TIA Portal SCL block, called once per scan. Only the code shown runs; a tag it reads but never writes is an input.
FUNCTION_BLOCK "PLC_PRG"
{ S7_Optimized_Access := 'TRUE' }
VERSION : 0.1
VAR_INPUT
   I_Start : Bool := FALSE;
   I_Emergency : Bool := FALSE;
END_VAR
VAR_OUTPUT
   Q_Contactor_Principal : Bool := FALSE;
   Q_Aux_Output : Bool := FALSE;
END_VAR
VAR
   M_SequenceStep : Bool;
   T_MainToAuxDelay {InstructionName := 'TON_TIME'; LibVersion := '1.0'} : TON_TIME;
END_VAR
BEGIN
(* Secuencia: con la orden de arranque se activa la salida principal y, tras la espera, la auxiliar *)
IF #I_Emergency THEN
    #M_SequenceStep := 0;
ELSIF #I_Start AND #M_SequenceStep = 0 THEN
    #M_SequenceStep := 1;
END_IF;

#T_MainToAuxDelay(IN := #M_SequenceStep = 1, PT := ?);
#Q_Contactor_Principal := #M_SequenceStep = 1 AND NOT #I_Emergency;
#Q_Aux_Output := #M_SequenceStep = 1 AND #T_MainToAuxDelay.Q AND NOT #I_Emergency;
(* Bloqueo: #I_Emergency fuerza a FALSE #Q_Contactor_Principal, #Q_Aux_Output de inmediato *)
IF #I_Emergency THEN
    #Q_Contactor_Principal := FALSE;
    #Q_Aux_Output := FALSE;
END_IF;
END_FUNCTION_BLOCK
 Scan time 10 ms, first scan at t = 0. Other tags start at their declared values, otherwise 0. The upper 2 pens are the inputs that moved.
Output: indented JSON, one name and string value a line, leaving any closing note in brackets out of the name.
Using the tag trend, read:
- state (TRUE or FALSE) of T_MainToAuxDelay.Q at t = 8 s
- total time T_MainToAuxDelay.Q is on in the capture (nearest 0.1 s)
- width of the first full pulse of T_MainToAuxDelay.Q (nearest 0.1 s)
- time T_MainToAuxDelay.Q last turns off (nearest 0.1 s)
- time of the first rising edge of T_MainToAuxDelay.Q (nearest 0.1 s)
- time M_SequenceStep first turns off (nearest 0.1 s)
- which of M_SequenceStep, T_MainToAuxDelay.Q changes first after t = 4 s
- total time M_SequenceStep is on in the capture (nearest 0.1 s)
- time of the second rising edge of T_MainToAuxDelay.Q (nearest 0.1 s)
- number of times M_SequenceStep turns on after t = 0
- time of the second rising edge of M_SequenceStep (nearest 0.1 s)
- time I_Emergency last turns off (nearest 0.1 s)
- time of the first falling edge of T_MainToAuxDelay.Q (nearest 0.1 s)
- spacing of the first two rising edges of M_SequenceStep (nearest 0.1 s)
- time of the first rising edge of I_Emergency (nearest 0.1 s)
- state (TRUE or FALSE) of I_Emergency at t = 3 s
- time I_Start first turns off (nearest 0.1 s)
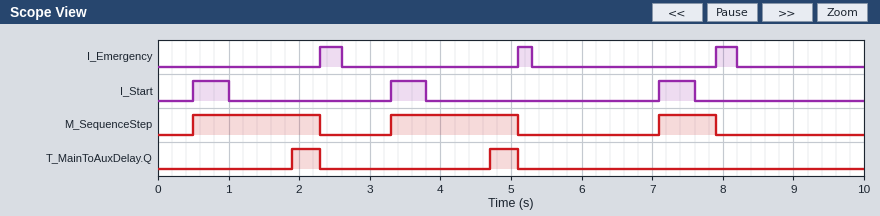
{
  "state (TRUE or FALSE) of T_MainToAuxDelay.Q at t = 8 s": "FALSE",
  "total time T_MainToAuxDelay.Q is on in the capture": "0.8 s",
  "width of the first full pulse of T_MainToAuxDelay.Q": "0.4 s",
  "time T_MainToAuxDelay.Q last turns off": "5.1 s",
  "time of the first rising edge of T_MainToAuxDelay.Q": "1.9 s",
  "time M_SequenceStep first turns off": "2.3 s",
  "which of M_SequenceStep, T_MainToAuxDelay.Q changes first after t = 4 s": "T_MainToAuxDelay.Q",
  "total time M_SequenceStep is on in the capture": "4.4 s",
  "time of the second rising edge of T_MainToAuxDelay.Q": "4.7 s",
  "number of times M_SequenceStep turns on after t = 0": "3",
  "time of the second rising edge of M_SequenceStep": "3.3 s",
  "time I_Emergency last turns off": "8.2 s",
  "time of the first falling edge of T_MainToAuxDelay.Q": "2.3 s",
  "spacing of the first two rising edges of M_SequenceStep": "2.8 s",
  "time of the first rising edge of I_Emergency": "2.3 s",
  "state (TRUE or FALSE) of I_Emergency at t = 3 s": "FALSE",
  "time I_Start first turns off": "1.0 s"
}
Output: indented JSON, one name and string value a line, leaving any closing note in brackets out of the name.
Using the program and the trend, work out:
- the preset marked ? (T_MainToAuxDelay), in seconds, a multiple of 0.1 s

{
  "the preset marked ? (T_MainToAuxDelay), in seconds, a multiple of 0.1 s": "1.4 s"
}
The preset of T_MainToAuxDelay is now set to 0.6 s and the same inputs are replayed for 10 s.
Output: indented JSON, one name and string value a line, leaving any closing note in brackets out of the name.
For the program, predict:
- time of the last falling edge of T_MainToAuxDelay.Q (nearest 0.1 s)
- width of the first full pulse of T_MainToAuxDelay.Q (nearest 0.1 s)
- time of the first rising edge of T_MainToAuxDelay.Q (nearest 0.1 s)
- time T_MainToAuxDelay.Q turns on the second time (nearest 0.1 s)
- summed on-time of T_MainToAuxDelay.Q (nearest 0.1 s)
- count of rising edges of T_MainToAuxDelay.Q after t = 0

{
  "time of the last falling edge of T_MainToAuxDelay.Q": "7.9 s",
  "width of the first full pulse of T_MainToAuxDelay.Q": "1.2 s",
  "time of the first rising edge of T_MainToAuxDelay.Q": "1.1 s",
  "time T_MainToAuxDelay.Q turns on the second time": "3.9 s",
  "summed on-time of T_MainToAuxDelay.Q": "2.6 s",
  "count of rising edges of T_MainToAuxDelay.Q after t = 0": "3"
}
